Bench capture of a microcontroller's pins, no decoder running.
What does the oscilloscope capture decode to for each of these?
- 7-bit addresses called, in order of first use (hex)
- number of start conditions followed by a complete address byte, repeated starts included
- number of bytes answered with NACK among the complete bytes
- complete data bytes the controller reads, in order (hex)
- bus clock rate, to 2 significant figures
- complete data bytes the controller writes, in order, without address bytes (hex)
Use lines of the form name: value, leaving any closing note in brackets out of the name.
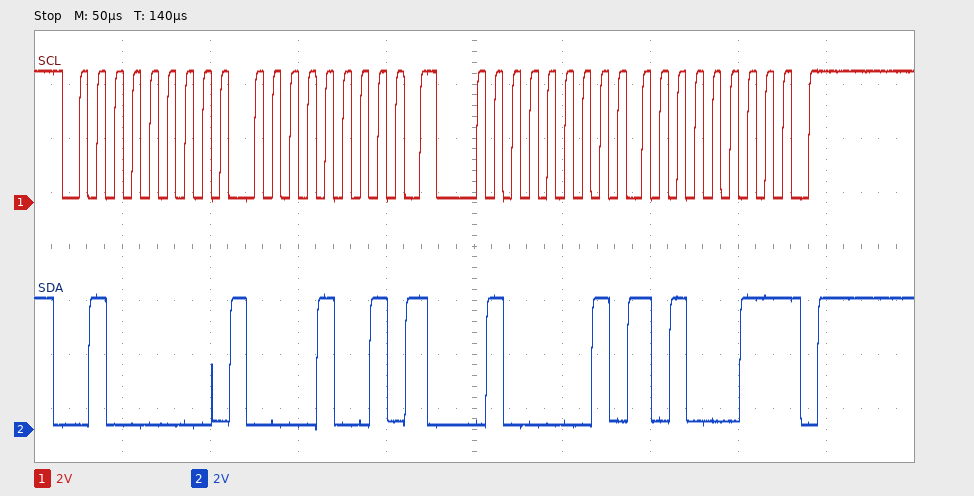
7-bit addresses called, in order of first use: 0x20
number of start conditions followed by a complete address byte, repeated starts included: 2
number of bytes answered with NACK among the complete bytes: 1
complete data bytes the controller reads, in order: A3
bus clock rate, to 2 significant figures: 100 kHz
complete data bytes the controller writes, in order, without address bytes: 09
